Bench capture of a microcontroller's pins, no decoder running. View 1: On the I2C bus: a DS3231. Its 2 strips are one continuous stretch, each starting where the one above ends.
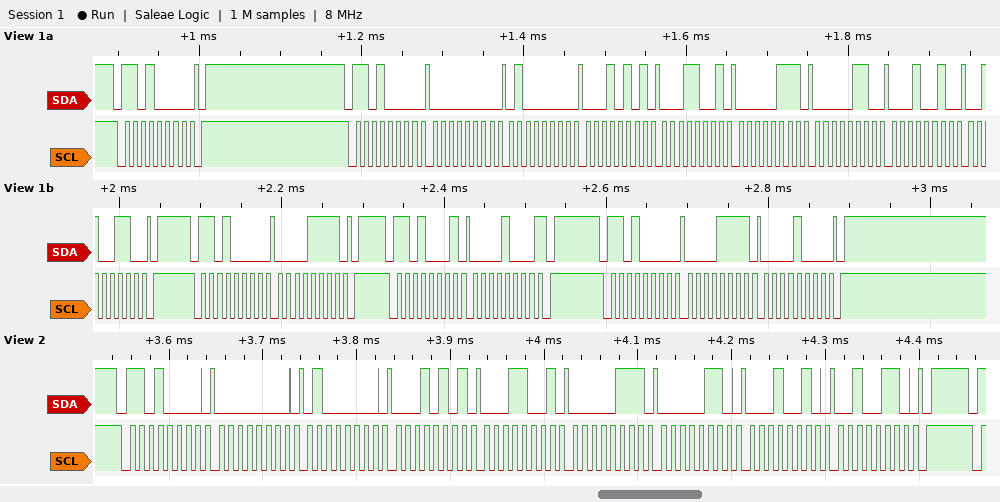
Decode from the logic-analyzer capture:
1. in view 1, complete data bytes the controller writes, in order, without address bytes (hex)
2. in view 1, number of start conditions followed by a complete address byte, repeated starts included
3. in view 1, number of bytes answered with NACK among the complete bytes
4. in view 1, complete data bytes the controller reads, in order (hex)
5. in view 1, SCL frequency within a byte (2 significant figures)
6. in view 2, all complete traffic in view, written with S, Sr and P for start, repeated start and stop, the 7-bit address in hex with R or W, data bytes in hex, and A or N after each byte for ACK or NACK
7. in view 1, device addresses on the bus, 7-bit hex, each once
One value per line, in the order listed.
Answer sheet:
00 40 15 19 07 06 12 26 0F 0F 08
5
1
08
100 kHz
S 68W A 00 A 40 A 15 A 19 A 07 A 06 A 12 A 26 A P
0x68
